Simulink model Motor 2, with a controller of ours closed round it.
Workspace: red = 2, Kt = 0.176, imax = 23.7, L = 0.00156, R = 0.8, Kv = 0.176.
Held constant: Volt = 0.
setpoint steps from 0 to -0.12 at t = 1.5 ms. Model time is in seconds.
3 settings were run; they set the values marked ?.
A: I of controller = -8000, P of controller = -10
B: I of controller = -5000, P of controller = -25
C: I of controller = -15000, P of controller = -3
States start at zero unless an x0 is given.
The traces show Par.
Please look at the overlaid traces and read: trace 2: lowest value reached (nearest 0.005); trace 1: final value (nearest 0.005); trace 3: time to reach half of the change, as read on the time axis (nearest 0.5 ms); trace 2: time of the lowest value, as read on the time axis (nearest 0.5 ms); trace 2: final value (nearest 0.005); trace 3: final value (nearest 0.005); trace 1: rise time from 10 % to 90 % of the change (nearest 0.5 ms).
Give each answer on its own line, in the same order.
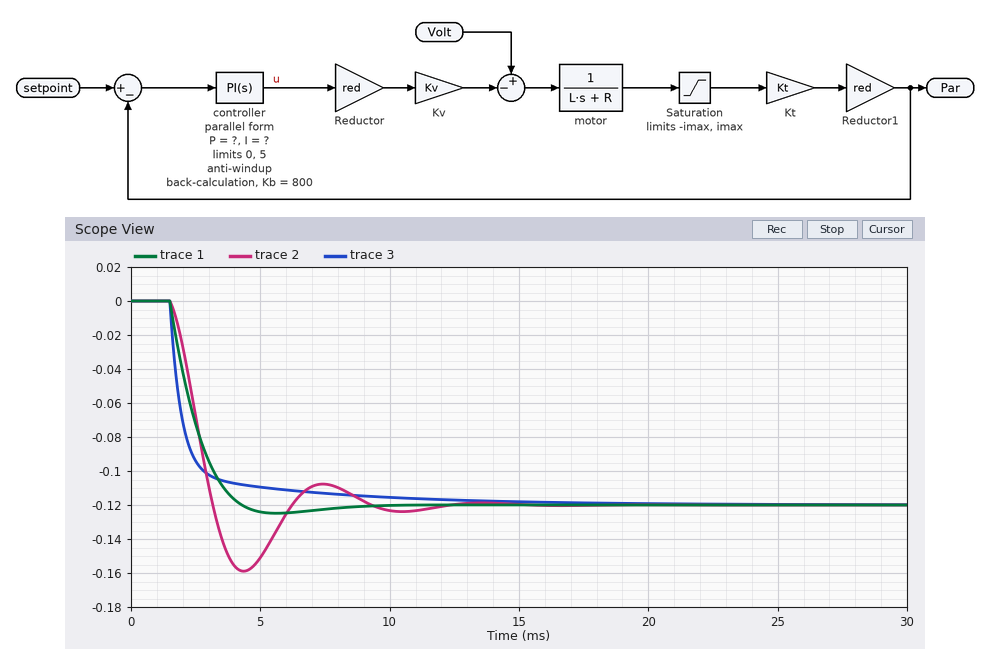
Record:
-0.160
-0.120
2.0 ms
4.5 ms
-0.120
-0.120
2.0 ms
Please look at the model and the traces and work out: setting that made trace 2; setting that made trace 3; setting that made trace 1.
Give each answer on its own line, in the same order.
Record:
C
B
A
